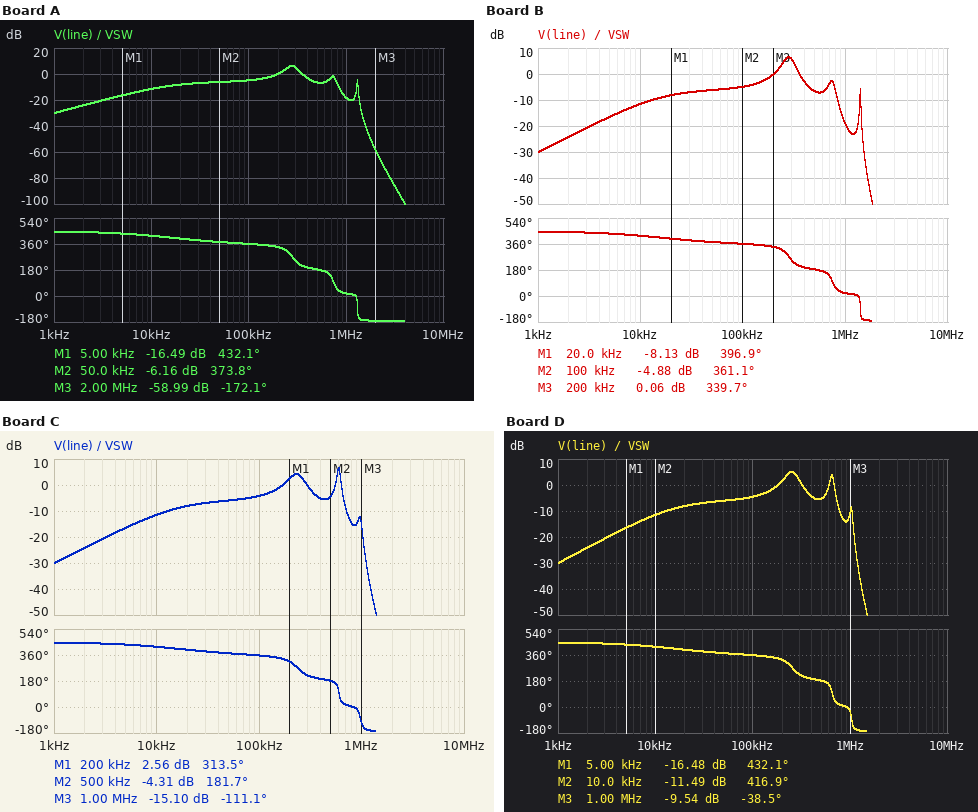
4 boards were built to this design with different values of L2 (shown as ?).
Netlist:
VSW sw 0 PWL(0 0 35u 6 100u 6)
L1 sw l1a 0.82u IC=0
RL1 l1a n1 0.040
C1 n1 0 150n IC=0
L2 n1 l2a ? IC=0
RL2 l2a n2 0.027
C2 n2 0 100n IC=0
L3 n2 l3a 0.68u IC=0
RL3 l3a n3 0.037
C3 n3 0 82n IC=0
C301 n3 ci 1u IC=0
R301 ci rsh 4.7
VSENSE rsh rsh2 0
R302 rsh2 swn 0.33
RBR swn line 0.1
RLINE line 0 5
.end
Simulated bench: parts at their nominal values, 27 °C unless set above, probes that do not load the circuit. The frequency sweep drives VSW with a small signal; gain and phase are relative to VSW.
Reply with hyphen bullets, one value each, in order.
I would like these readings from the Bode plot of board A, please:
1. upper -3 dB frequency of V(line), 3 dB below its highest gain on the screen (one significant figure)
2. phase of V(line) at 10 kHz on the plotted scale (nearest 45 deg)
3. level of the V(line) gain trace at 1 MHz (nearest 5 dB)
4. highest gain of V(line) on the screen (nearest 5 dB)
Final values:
- 300 kHz
- 405 deg
- -20 dB
- 5 dB
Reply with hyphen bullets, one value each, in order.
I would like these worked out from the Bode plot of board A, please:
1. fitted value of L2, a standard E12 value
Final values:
- 330 nH
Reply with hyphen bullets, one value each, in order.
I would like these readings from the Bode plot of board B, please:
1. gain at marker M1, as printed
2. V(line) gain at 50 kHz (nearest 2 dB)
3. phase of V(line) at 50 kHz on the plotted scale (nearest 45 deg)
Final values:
- -8.13 dB
- -6 dB
- 360 deg
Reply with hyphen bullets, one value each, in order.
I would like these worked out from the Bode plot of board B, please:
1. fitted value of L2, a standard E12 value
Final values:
- 270 nH
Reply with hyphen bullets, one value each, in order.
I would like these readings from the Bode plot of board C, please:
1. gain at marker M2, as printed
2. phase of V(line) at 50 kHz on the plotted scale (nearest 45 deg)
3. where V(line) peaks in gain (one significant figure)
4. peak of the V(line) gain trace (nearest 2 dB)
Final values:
- -4.31 dB
- 360 deg
- 600 kHz
- 6 dB
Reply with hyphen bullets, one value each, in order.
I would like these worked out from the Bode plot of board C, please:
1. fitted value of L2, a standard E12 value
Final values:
- 1.2 µH
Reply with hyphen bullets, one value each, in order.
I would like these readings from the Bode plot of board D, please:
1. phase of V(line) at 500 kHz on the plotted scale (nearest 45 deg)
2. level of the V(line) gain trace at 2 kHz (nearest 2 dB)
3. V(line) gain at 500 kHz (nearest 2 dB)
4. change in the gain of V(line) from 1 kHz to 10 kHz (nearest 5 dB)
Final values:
- 180 deg
- -24 dB
- -6 dB
- 20 dB
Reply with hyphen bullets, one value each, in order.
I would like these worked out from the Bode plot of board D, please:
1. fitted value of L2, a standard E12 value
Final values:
- 820 nH
